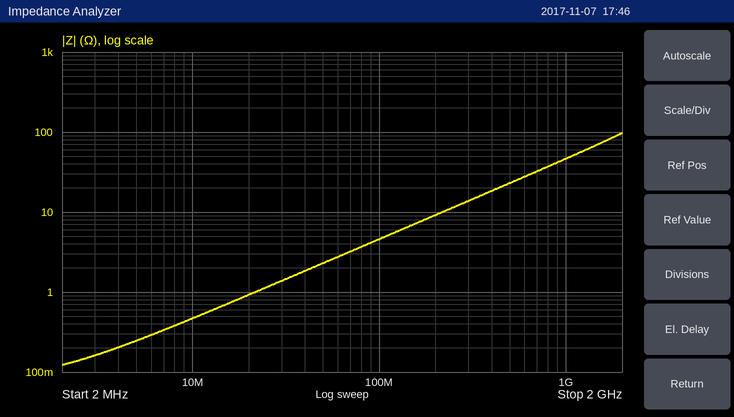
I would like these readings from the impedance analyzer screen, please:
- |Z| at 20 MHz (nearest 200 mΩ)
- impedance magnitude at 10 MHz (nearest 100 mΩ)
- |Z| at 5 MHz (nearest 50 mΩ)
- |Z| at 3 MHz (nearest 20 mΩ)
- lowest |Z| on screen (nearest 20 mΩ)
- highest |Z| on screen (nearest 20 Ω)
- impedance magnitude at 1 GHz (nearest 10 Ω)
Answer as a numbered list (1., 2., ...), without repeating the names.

1. 1.0 Ω
2. 500 mΩ
3. 250 mΩ
4. 160 mΩ
5. 120 mΩ
6. 100 Ω
7. 50 Ω
